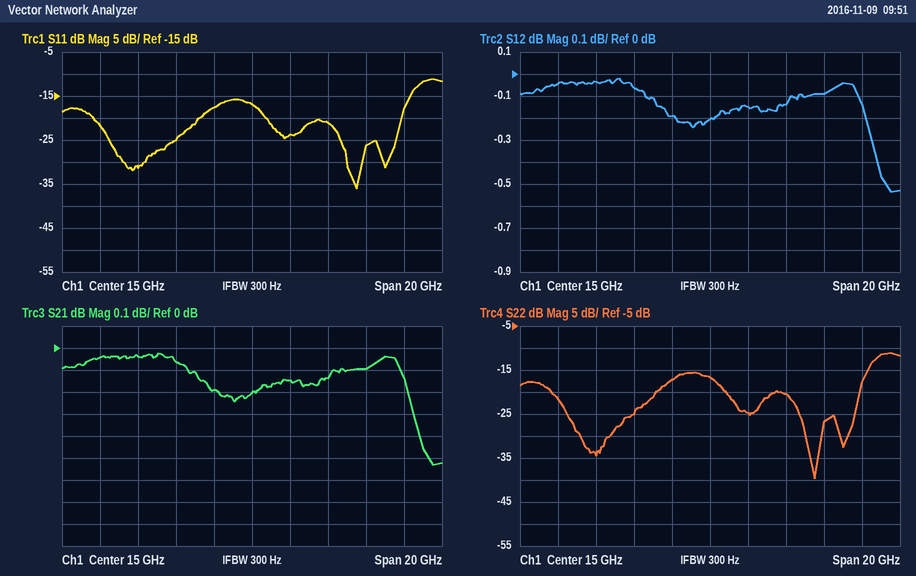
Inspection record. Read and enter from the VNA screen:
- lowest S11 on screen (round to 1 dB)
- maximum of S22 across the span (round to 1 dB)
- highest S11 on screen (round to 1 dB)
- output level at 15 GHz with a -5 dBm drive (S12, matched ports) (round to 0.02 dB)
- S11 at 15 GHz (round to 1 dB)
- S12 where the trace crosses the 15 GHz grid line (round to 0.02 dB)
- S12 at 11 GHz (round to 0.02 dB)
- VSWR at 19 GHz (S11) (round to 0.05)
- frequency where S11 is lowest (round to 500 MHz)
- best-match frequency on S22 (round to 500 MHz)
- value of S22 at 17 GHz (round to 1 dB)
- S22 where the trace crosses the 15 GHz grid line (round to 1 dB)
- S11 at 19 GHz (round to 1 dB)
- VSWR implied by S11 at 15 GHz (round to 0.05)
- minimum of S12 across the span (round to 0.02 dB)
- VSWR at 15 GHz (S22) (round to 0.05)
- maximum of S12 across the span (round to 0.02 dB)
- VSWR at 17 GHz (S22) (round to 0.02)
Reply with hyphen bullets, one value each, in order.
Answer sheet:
- -36 dB
- -11 dB
- -11 dB
- -5.20 dBm
- -17 dB
- -0.20 dB
- -0.06 dB
- 1.20
- 20.5 GHz
- 20.5 GHz
- -25 dB
- -17 dB
- -21 dB
- 1.35
- -0.54 dB
- 1.35
- -0.02 dB
- 1.12
